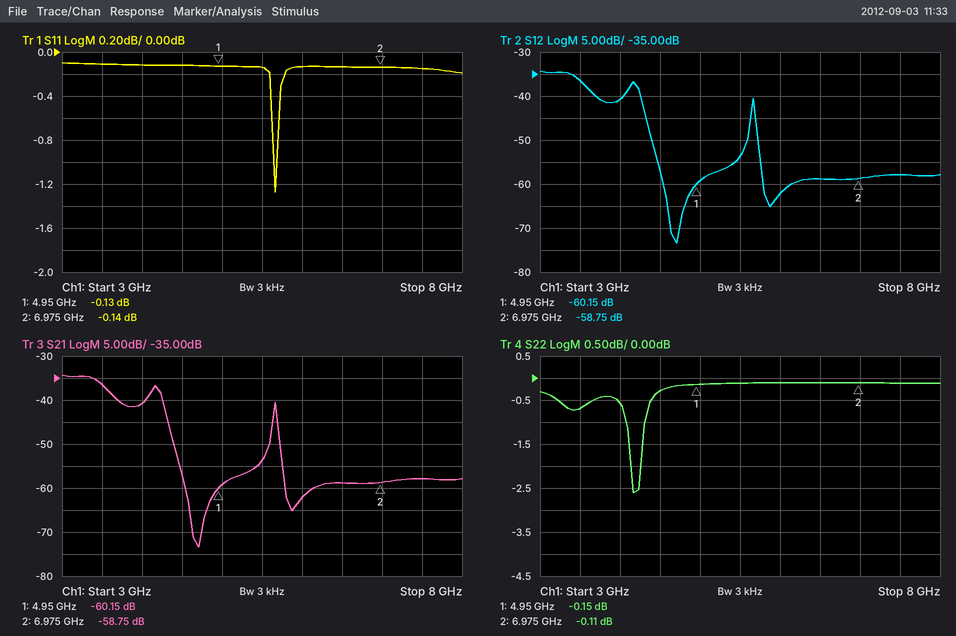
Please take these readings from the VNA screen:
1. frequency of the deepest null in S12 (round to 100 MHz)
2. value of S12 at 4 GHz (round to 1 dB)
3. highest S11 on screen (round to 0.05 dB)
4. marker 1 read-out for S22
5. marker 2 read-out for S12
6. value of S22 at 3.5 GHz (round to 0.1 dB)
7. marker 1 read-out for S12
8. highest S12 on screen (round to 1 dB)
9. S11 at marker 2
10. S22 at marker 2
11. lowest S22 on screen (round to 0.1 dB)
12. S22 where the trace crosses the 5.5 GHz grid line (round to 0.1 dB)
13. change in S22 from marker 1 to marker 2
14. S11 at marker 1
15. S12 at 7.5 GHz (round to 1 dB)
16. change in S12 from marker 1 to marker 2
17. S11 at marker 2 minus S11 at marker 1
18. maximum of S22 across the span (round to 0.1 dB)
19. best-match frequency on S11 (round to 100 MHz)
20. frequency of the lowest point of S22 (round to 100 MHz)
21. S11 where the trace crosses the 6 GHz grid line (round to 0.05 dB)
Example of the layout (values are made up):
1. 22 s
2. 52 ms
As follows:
1. 4.7 GHz
2. -41 dB
3. -0.10 dB
4. -0.15 dB
5. -58.75 dB
6. -0.7 dB
7. -60.15 dB
8. -34 dB
9. -0.14 dB
10. -0.11 dB
11. -2.6 dB
12. -0.1 dB
13. 0.04 dB
14. -0.13 dB
15. -58 dB
16. 1.40 dB
17. -0.01 dB
18. -0.1 dB
19. 5.7 GHz
20. 4.2 GHz
21. -0.15 dB
